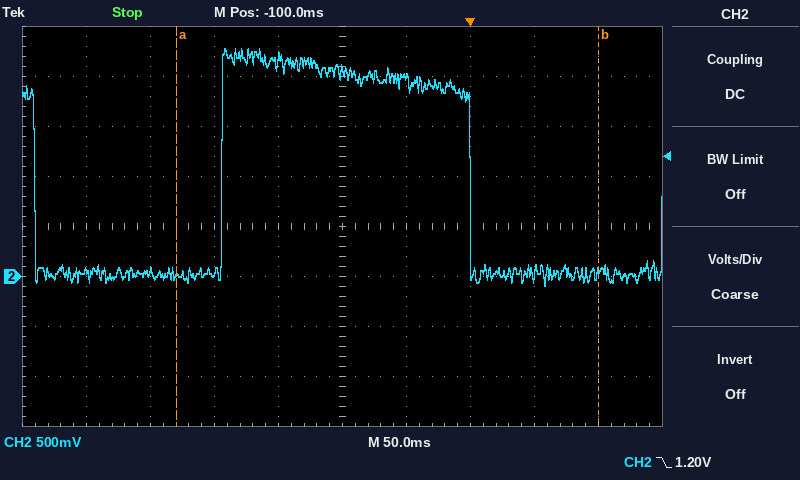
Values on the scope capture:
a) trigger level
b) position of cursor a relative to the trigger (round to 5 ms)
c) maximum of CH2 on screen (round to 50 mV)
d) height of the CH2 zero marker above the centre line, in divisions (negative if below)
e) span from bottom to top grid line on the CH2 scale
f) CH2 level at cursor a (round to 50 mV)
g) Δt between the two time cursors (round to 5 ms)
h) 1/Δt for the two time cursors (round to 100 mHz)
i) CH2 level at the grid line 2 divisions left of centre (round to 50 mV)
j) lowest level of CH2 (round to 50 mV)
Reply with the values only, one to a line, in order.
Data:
1.20 V
-230 ms
2.30 V
-1.0 div
4 V
0 mV
330 ms
3.0 Hz
50 mV
-100 mV
